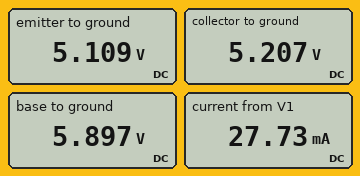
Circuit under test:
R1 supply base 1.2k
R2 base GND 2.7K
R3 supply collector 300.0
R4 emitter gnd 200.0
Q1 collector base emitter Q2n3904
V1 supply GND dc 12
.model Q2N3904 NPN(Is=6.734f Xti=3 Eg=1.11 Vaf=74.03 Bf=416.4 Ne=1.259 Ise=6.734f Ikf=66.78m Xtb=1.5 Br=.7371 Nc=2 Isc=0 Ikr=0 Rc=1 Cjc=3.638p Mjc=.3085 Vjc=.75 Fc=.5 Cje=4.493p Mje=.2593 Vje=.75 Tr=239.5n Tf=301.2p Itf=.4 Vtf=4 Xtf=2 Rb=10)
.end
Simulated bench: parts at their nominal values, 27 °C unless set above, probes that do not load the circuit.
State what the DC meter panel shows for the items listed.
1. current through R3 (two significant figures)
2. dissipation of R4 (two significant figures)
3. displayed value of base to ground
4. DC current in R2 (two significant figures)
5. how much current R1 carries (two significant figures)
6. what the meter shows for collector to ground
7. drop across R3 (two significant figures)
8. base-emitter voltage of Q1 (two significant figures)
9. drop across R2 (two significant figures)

23 mA
130 mW
5.897 V
2.2 mA
5.1 mA
5.207 V
6.8 V
790 mV
5.9 V
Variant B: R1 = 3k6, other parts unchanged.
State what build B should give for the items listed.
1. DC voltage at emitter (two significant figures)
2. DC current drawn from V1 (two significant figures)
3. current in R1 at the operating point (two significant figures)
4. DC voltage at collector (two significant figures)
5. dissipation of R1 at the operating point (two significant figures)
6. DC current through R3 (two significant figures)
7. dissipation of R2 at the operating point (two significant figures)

4.2 V
23 mA
2.0 mA
5.8 V
14 mW
21 mA
9.0 mW
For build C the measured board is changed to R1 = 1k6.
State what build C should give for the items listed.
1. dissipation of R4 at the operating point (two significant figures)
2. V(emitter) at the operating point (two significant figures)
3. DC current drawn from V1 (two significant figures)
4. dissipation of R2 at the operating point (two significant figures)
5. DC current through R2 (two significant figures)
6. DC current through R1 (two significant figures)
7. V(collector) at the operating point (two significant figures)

120 mW
5.0 V
27 mA
12 mW
2.1 mA
3.9 mA
5.1 V
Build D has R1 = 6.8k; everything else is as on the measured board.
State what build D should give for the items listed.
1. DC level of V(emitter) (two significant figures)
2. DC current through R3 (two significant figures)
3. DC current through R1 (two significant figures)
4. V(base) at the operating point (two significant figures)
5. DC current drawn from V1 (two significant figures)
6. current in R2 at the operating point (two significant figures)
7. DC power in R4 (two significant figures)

2.5 V
13 mA
1.3 mA
3.3 V
14 mA
1.2 mA
32 mW
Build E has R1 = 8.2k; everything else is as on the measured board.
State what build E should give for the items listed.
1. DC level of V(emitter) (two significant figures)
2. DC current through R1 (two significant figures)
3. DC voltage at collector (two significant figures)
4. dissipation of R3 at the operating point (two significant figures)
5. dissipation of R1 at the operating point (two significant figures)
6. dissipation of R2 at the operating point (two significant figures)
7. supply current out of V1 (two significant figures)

2.1 V
1.1 mA
8.8 V
33 mW
10 mW
3.0 mW
12 mA
